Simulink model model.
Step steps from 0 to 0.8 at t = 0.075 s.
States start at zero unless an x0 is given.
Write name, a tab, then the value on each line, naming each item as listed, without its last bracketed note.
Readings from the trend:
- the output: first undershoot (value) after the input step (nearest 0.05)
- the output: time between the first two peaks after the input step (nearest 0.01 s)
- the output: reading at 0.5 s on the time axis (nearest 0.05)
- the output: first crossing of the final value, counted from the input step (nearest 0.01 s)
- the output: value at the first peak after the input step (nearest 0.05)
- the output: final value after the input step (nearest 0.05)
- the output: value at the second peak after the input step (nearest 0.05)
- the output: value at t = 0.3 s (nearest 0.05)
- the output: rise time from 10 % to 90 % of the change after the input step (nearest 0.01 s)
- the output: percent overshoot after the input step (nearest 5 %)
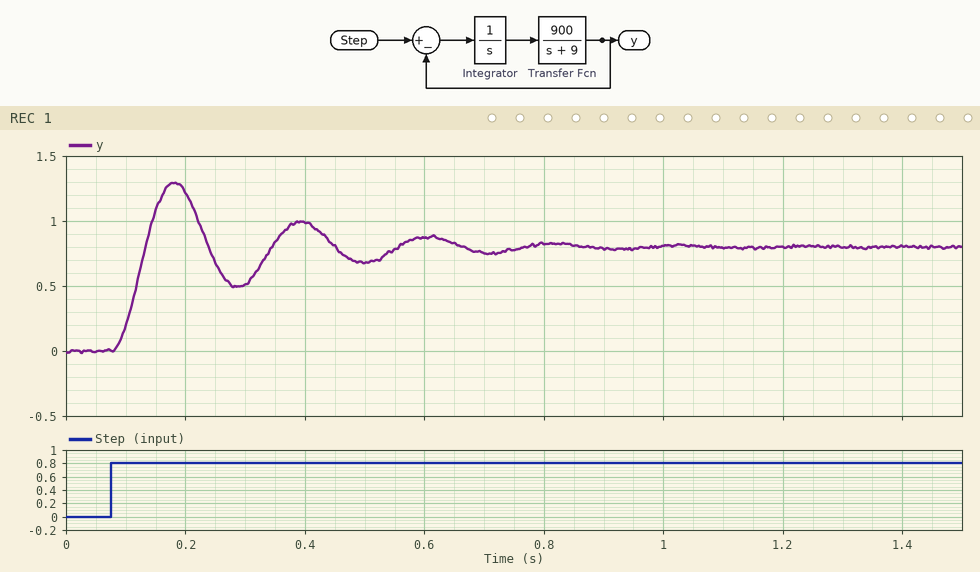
the output: first undershoot (value) after the input step	0.50
the output: time between the first two peaks after the input step	0.21 s
the output: reading at 0.5 s on the time axis	0.70
the output: first crossing of the final value, counted from the input step	0.06 s
the output: value at the first peak after the input step	1.30
the output: final value after the input step	0.80
the output: value at the second peak after the input step	1.00
the output: value at t = 0.3 s	0.50
the output: rise time from 10 % to 90 % of the change after the input step	0.04 s
the output: percent overshoot after the input step	60 %
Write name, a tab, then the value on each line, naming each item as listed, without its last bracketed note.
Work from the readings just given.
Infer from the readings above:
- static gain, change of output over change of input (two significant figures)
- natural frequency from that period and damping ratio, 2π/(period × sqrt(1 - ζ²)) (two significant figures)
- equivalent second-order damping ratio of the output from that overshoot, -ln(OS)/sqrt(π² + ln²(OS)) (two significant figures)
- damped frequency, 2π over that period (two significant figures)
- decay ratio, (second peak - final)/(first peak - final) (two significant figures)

static gain, change of output over change of input	1.0
natural frequency from that period and damping ratio, 2π/(period × sqrt(1 - ζ²))	30 rad/s
equivalent second-order damping ratio of the output from that overshoot, -ln(OS)/sqrt(π² + ln²(OS))	0.16
damped frequency, 2π over that period	30 rad/s
decay ratio, (second peak - final)/(first peak - final)	0.40
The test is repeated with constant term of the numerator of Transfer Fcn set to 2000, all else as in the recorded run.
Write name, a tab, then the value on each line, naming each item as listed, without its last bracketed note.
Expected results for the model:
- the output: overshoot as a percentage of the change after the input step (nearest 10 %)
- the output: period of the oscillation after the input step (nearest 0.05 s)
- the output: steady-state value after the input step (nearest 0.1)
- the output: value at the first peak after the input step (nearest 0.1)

the output: overshoot as a percentage of the change after the input step	70 %
the output: period of the oscillation after the input step	0.15 s
the output: steady-state value after the input step	0.8
the output: value at the first peak after the input step	1.4
